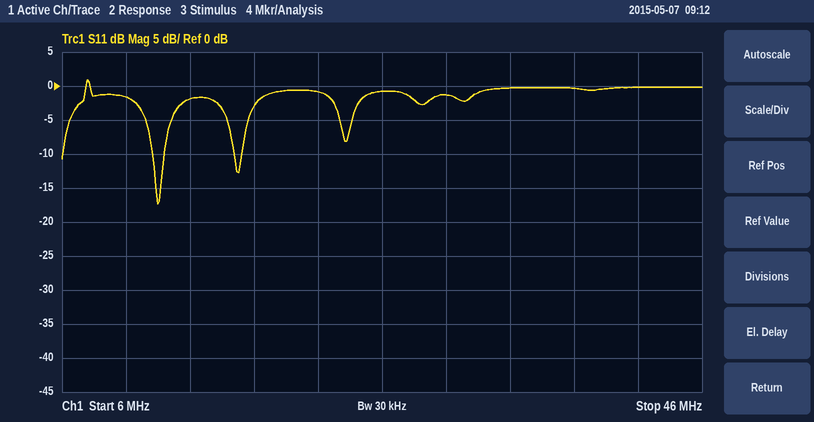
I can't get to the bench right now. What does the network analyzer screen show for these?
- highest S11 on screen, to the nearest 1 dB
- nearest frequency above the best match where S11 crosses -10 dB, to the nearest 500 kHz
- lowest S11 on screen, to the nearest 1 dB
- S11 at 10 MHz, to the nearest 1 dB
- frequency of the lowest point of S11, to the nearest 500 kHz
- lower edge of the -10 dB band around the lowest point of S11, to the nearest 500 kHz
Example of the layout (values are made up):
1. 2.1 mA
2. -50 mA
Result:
1. 1 dB
2. 12.5 MHz
3. -17 dB
4. -2 dB
5. 12.0 MHz
6. 11.5 MHz
